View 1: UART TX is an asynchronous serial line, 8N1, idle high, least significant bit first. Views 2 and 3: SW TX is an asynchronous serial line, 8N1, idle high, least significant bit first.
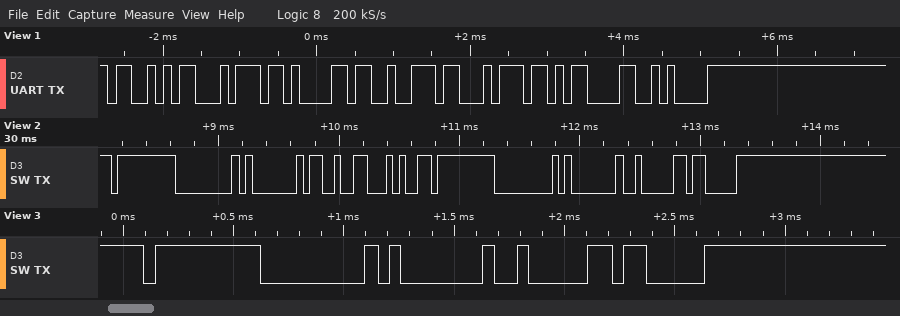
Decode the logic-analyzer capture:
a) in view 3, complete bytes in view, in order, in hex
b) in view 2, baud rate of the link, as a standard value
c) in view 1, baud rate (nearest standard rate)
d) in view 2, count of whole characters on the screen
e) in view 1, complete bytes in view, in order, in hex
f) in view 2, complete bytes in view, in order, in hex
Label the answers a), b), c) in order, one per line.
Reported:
a) FF 00 01 82 83
b) 19200 baud
c) 9600 baud
d) 10
e) 53 74 61 72 74 0D 0A
f) FF 00 01 93 94 FF 00 01 82 83
